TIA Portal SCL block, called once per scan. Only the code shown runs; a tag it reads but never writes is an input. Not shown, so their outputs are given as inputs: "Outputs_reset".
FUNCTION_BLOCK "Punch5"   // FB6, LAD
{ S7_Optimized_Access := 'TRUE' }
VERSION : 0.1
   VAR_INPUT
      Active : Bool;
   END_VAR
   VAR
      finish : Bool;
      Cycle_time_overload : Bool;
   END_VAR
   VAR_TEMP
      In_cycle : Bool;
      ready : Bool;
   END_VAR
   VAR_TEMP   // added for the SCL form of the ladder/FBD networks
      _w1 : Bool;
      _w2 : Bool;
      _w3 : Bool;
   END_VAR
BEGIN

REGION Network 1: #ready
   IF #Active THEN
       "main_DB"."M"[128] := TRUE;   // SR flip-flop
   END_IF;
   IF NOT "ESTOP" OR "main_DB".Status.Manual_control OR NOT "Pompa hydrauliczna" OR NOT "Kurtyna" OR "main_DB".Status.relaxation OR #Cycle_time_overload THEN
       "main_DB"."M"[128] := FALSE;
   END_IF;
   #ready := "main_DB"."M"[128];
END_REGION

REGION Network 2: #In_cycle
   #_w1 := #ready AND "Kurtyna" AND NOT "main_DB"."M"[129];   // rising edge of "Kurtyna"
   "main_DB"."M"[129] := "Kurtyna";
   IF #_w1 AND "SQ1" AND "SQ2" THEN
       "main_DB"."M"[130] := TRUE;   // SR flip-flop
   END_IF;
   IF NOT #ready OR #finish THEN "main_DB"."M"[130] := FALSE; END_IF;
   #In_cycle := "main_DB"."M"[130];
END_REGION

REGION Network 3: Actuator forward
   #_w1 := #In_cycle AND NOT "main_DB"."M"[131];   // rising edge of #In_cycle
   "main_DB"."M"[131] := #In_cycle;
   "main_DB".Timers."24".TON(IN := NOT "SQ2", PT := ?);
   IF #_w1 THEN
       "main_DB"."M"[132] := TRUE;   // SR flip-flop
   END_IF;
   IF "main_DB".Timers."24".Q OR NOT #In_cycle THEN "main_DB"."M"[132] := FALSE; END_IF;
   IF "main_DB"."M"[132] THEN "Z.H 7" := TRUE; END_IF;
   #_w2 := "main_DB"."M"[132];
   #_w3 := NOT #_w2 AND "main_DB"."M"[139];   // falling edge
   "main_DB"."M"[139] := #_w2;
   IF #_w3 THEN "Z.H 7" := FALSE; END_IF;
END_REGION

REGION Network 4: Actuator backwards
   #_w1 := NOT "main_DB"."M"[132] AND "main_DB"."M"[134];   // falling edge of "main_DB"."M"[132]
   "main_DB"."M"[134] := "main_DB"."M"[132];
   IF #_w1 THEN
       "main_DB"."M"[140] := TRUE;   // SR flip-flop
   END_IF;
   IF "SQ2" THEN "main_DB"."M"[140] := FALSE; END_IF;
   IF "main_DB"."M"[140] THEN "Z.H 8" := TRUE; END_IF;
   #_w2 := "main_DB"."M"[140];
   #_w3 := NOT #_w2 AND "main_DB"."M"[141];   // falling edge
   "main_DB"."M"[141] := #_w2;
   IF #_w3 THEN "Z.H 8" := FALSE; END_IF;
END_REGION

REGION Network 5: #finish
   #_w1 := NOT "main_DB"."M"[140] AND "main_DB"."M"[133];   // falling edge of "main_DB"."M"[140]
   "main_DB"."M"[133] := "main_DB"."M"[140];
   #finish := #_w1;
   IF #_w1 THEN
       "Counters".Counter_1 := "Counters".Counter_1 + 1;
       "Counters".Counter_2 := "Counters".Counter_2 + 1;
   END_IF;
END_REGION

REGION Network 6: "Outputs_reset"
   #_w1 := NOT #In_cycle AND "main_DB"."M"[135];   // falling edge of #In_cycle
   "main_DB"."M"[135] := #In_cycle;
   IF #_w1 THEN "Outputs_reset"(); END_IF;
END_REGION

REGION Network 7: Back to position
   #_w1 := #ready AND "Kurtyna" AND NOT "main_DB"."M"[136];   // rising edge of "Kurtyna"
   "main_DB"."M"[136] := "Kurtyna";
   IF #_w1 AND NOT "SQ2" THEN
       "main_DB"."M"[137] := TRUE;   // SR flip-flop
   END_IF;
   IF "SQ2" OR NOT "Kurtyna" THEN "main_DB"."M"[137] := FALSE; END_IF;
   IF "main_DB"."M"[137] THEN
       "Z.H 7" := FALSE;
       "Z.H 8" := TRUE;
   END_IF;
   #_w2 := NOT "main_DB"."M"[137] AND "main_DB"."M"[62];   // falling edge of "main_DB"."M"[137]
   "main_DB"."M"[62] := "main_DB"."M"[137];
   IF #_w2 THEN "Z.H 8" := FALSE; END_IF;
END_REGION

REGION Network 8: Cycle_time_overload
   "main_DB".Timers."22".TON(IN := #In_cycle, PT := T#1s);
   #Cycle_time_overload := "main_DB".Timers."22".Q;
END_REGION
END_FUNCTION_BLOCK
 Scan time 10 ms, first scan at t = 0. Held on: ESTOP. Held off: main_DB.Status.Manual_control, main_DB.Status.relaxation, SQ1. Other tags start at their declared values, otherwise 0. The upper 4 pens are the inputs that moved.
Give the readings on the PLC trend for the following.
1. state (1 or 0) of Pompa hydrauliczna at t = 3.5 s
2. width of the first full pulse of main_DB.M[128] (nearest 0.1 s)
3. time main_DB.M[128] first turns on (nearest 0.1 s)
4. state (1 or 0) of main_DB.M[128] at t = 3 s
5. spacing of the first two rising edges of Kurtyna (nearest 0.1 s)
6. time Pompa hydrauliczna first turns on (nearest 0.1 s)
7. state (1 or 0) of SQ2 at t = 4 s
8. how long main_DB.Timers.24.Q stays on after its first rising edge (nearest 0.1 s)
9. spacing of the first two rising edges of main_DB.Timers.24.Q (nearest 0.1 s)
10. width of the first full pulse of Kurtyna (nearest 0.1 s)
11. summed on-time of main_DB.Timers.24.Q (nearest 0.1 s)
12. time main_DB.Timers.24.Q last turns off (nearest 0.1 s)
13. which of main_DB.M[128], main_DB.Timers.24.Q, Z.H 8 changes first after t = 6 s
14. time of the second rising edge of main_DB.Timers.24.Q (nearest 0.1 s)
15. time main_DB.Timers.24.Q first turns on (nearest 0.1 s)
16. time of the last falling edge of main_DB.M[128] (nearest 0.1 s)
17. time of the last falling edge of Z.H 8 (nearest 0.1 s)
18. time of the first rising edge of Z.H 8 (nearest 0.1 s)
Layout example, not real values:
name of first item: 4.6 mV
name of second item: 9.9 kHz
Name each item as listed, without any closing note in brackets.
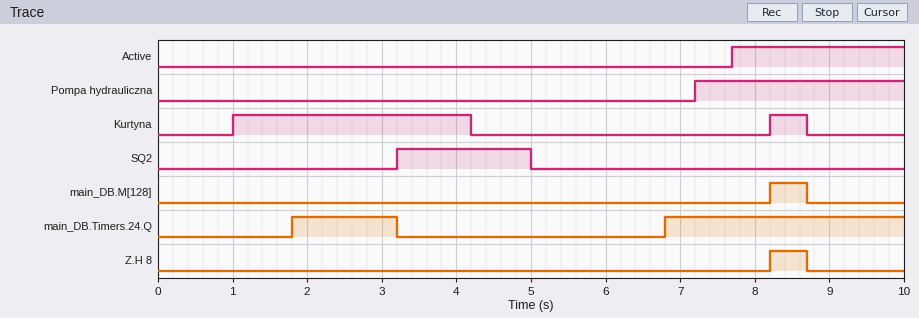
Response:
state (1 or 0) of Pompa hydrauliczna at t = 3.5 s: 0
width of the first full pulse of main_DB.M[128]: 0.5 s
time main_DB.M[128] first turns on: 8.2 s
state (1 or 0) of main_DB.M[128] at t = 3 s: 0
spacing of the first two rising edges of Kurtyna: 7.2 s
time Pompa hydrauliczna first turns on: 7.2 s
state (1 or 0) of SQ2 at t = 4 s: 1
how long main_DB.Timers.24.Q stays on after its first rising edge: 1.4 s
spacing of the first two rising edges of main_DB.Timers.24.Q: 5.0 s
width of the first full pulse of Kurtyna: 3.2 s
summed on-time of main_DB.Timers.24.Q: 4.6 s
time main_DB.Timers.24.Q last turns off: 3.2 s
which of main_DB.M[128], main_DB.Timers.24.Q, Z.H 8 changes first after t = 6 s: main_DB.Timers.24.Q
time of the second rising edge of main_DB.Timers.24.Q: 6.8 s
time main_DB.Timers.24.Q first turns on: 1.8 s
time of the last falling edge of main_DB.M[128]: 8.7 s
time of the last falling edge of Z.H 8: 8.7 s
time of the first rising edge of Z.H 8: 8.2 s
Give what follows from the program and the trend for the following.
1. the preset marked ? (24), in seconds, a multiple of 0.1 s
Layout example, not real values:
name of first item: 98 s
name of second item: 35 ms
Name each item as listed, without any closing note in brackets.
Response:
the preset marked ? (24), in seconds, a multiple of 0.1 s: 1.8 s
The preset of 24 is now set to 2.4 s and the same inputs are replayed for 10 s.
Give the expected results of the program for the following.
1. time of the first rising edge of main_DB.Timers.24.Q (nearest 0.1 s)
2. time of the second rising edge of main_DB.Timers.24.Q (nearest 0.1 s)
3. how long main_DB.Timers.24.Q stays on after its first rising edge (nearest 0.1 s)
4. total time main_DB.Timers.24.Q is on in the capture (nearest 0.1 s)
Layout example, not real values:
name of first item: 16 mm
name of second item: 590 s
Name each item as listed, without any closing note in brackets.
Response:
time of the first rising edge of main_DB.Timers.24.Q: 2.4 s
time of the second rising edge of main_DB.Timers.24.Q: 7.4 s
how long main_DB.Timers.24.Q stays on after its first rising edge: 0.8 s
total time main_DB.Timers.24.Q is on in the capture: 3.4 s
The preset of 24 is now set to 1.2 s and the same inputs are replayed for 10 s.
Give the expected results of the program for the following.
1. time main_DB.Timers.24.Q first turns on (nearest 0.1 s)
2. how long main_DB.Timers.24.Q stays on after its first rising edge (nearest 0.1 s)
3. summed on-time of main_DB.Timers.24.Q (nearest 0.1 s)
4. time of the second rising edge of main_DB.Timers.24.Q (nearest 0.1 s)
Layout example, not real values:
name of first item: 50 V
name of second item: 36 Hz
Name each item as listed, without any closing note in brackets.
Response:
time main_DB.Timers.24.Q first turns on: 1.2 s
how long main_DB.Timers.24.Q stays on after its first rising edge: 2.0 s
summed on-time of main_DB.Timers.24.Q: 5.8 s
time of the second rising edge of main_DB.Timers.24.Q: 6.2 s
